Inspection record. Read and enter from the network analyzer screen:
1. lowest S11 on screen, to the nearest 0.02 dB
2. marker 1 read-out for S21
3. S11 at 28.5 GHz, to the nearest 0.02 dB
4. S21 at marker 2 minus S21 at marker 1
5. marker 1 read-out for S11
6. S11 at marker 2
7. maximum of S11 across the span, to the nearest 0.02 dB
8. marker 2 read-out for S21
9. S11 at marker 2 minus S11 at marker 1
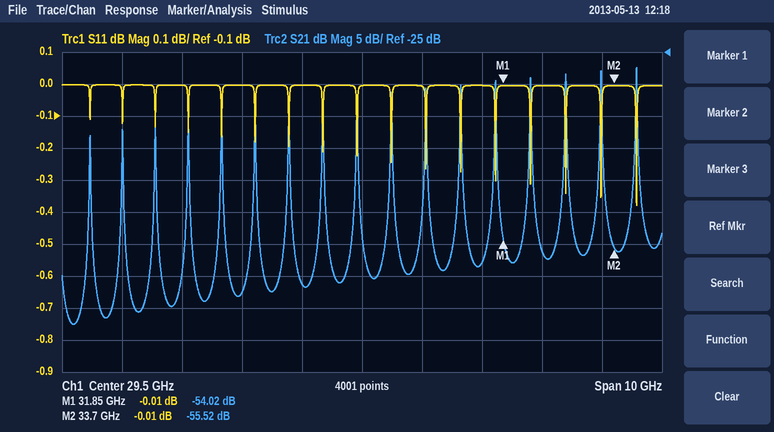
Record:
-0.38 dB
-54.02 dB
0.00 dB
-1.50 dB
-0.01 dB
-0.01 dB
0.00 dB
-55.52 dB
0.00 dB
